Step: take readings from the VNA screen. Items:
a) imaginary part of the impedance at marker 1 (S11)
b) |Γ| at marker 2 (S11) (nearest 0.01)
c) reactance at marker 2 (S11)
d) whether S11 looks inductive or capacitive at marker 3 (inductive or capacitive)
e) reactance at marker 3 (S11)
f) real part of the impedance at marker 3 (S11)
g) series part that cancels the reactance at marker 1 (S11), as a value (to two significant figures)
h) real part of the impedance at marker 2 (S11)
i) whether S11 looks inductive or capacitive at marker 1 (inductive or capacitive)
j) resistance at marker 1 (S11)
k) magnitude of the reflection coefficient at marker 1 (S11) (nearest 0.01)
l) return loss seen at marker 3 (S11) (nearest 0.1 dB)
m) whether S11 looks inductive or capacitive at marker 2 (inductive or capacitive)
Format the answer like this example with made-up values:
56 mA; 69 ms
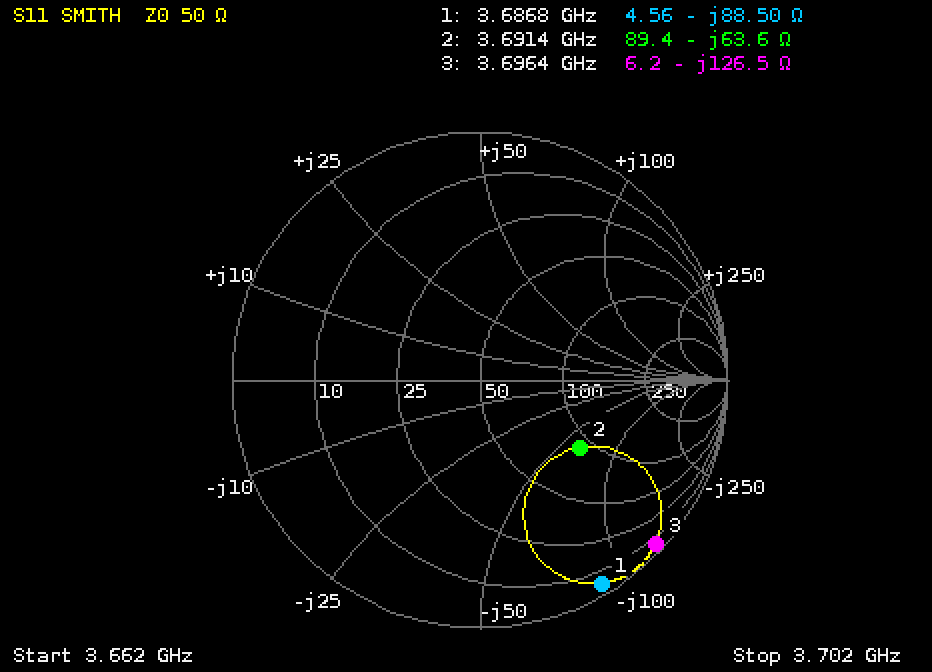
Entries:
-88.50 Ω; 0.49; -63.6 Ω; capacitive; -126.5 Ω; 6.2 Ω; 3.8 nH; 89.4 Ω; capacitive; 4.56 Ω; 0.96; 0.3 dB; capacitive
